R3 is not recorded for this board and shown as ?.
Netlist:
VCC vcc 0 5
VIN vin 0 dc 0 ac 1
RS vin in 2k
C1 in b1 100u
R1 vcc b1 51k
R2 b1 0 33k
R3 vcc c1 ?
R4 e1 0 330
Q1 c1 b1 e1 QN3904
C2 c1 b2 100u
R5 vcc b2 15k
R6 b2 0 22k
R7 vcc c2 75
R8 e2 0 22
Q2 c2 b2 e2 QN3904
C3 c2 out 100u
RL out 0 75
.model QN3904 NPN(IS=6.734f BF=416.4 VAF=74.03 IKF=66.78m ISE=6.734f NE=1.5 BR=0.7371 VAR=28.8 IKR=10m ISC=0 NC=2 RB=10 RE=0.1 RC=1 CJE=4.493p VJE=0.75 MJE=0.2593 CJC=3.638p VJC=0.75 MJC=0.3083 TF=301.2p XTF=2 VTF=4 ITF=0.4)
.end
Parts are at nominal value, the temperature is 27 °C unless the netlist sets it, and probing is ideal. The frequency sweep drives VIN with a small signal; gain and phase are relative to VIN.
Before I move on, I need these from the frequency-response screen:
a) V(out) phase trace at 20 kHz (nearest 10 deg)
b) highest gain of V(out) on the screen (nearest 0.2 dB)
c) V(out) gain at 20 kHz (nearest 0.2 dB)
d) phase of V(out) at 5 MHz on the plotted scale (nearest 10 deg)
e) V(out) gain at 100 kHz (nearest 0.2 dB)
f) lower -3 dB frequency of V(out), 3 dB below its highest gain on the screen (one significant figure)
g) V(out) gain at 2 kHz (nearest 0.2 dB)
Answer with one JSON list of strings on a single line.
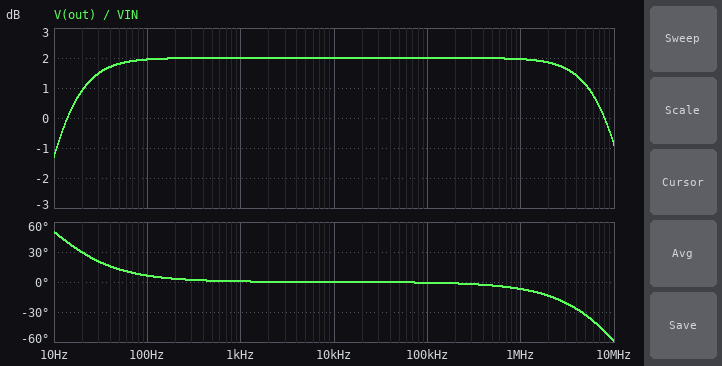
["0 deg", "2.0 dB", "2.0 dB", "-30 deg", "2.0 dB", "10 Hz", "2.0 dB"]
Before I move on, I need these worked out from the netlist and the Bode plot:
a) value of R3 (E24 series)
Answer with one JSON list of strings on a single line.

["330 Ω"]
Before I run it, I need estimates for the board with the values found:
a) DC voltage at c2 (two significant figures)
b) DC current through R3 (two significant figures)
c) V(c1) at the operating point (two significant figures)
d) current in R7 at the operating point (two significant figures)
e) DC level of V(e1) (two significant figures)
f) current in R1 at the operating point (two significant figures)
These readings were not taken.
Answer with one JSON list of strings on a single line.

["2.1 V", "3.3 mA", "3.9 V", "38 mA", "1.1 V", "63 µA"]
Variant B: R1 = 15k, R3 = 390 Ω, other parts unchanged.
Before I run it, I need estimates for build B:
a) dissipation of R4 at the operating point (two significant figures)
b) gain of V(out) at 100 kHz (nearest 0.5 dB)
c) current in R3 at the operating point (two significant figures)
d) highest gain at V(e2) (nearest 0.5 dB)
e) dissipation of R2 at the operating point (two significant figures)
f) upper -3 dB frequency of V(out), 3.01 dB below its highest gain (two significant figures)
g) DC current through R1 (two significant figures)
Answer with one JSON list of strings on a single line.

["15 mW", "-15.5 dB", "6.7 mA", "-20.0 dB", "260 µW", "27 MHz", "140 µA"]
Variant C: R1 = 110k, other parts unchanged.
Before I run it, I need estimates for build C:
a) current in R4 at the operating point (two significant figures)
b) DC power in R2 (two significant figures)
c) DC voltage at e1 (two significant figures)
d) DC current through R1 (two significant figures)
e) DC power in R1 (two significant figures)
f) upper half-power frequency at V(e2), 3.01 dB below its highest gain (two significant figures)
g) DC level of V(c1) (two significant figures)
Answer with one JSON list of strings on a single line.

["1.2 mA", "35 µW", "400 mV", "36 µA", "140 µW", "11 MHz", "4.6 V"]
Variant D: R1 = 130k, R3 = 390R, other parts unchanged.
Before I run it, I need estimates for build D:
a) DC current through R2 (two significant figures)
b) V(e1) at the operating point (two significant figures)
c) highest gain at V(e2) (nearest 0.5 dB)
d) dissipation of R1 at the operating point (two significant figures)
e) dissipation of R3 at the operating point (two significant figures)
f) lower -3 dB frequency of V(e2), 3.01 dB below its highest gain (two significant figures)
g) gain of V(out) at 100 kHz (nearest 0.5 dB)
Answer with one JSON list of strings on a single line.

["29 µA", "290 mV", "-1.5 dB", "130 µW", "300 µW", "510 mHz", "3.0 dB"]
